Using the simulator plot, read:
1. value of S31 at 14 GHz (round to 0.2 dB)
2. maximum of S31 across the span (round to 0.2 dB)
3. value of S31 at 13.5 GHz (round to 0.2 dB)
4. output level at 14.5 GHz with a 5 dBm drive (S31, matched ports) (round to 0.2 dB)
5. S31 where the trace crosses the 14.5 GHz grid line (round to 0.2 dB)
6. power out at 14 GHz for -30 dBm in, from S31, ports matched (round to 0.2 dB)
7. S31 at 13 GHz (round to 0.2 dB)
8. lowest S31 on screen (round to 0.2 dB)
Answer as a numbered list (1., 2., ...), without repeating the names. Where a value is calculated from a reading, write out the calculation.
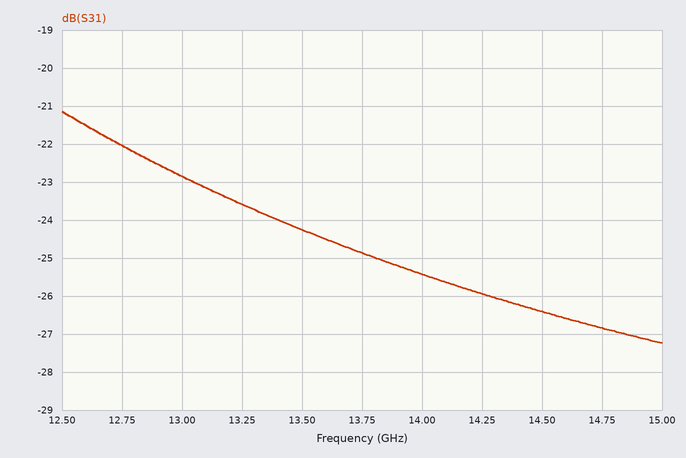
1. -25.4 dB
2. -21.2 dB
3. -24.2 dB
4. 5 dBm + (-26.4 dB) = -21.4 dBm
5. -26.4 dB
6. -30 dBm + (-25.4 dB) = -55.4 dBm
7. -22.8 dB
8. -27.2 dB
